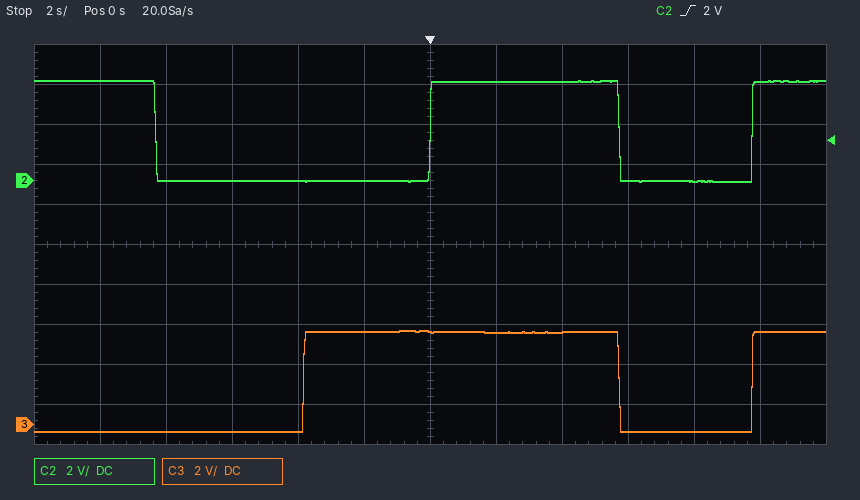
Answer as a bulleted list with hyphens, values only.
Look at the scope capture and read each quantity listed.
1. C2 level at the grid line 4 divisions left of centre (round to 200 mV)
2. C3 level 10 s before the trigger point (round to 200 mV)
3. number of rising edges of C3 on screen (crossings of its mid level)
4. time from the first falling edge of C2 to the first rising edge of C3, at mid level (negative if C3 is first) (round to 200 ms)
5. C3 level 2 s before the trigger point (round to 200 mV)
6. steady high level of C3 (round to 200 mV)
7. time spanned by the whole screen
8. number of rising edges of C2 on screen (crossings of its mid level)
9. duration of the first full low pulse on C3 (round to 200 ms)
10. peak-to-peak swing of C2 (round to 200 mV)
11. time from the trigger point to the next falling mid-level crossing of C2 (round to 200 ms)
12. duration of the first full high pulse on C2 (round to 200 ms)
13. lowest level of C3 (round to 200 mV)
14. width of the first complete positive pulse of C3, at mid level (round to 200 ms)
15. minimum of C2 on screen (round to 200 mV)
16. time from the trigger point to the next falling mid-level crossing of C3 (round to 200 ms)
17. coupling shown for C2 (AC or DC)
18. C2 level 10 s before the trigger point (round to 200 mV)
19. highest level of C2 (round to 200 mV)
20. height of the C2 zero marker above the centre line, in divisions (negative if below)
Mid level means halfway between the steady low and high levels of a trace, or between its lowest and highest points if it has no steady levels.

- 0.0 V
- -400 mV
- 2
- +4.4 s
- 4.6 V
- 4.6 V
- 24 s
- 2
- 4.0 s
- 5.0 V
- 5.8 s
- 5.8 s
- -400 mV
- 9.6 s
- 0.0 V
- 5.8 s
- DC
- 5.0 V
- 5.0 V
- +1.6 div
